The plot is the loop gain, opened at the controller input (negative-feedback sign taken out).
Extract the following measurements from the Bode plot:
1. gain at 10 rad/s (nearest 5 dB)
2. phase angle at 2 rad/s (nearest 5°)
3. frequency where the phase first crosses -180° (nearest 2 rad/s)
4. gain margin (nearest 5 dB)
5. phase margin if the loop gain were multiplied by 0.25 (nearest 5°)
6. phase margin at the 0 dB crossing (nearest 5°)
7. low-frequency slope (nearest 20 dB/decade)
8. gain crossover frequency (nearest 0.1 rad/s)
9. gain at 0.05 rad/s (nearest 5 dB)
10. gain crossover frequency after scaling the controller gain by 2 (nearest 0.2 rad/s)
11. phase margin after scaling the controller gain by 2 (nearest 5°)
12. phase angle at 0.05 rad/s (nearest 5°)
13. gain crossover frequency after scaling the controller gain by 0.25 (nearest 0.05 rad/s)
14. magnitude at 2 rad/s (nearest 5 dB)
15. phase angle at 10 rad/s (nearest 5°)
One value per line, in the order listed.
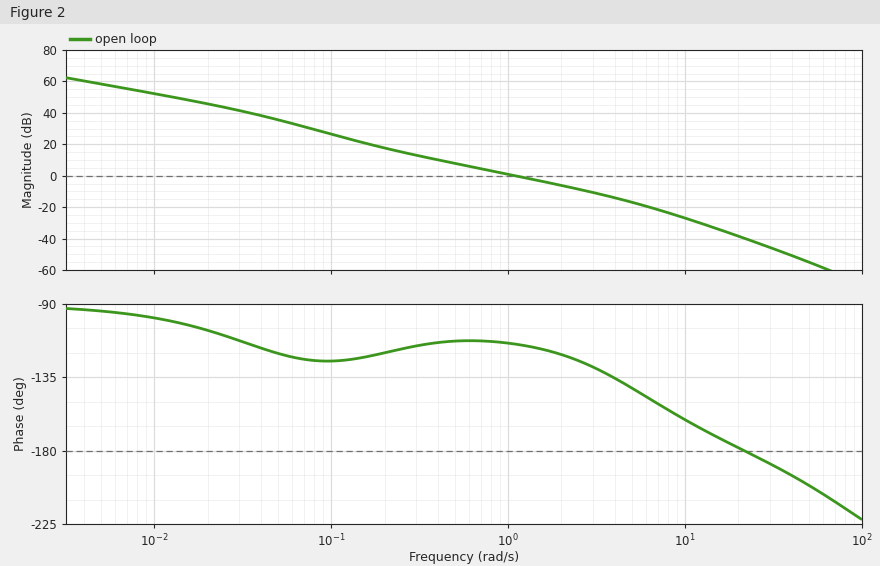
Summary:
-25 dB
-120°
22 rad/s
40 dB
65°
65°
-20 dB/decade
1.1 rad/s
35 dB
2.0 rad/s
60°
-120°
0.35 rad/s
-5 dB
-160°
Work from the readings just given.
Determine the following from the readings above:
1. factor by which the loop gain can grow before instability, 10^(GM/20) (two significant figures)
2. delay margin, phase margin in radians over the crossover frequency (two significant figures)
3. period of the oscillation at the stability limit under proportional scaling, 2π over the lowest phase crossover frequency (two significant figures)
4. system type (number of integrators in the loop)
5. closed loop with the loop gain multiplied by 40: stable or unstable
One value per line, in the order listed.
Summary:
100
1.0 s
0.29 s
1
stable
